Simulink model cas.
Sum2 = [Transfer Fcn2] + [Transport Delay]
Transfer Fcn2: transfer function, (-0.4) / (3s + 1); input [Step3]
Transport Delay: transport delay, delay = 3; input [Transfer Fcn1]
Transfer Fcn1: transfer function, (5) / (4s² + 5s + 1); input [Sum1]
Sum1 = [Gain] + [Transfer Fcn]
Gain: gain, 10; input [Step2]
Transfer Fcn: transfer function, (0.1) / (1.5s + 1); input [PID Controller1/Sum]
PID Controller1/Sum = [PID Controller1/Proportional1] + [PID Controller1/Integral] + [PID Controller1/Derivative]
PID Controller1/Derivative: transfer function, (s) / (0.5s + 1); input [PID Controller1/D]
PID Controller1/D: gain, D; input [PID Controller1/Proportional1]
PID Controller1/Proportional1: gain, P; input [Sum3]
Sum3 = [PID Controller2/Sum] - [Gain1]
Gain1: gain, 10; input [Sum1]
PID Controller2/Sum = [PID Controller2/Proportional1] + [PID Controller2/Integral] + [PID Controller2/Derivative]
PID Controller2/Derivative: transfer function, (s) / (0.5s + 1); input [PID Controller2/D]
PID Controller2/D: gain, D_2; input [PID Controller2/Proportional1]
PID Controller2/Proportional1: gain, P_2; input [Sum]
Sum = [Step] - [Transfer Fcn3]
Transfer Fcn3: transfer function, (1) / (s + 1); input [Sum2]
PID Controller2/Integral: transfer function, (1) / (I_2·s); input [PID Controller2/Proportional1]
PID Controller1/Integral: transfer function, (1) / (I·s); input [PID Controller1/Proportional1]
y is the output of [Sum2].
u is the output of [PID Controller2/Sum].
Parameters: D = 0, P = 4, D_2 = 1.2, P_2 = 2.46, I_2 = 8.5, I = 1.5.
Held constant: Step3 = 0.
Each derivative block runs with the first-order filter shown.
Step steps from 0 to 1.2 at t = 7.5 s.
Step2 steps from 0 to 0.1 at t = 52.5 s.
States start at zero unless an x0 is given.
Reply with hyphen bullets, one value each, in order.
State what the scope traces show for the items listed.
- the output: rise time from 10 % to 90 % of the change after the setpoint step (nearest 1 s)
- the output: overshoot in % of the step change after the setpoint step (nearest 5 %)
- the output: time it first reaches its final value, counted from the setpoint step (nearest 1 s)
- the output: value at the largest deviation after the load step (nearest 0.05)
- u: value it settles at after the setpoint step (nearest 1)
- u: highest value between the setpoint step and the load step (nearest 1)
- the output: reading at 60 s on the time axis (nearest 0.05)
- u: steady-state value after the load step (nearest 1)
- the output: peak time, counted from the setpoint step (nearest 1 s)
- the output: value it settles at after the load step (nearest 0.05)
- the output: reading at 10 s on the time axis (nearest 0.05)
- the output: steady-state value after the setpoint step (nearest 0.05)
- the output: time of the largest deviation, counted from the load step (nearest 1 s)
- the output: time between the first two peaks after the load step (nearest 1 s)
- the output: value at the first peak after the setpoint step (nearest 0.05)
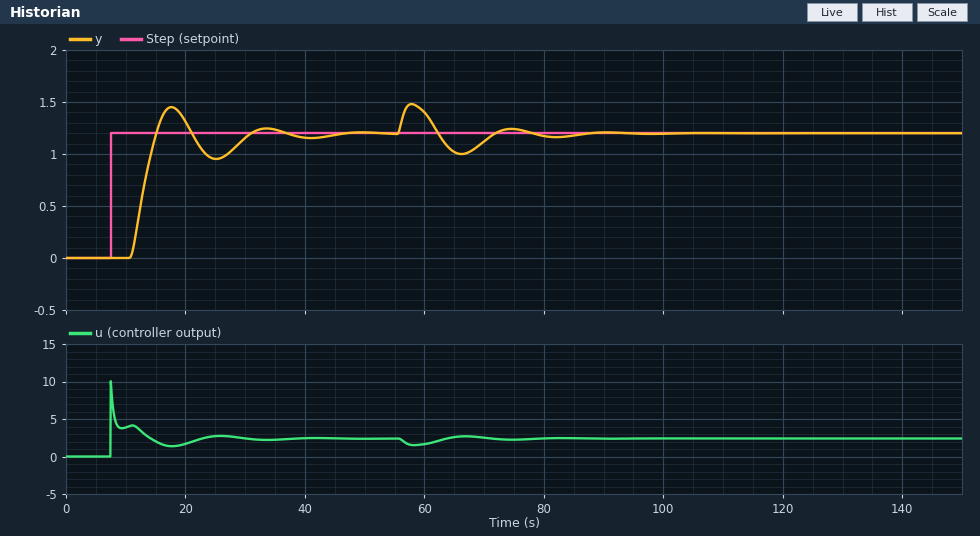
- 3 s
- 20 %
- 8 s
- 1.50
- 2
- 10
- 1.40
- 2
- 10 s
- 1.20
- 0.00
- 1.20
- 5 s
- 17 s
- 1.45
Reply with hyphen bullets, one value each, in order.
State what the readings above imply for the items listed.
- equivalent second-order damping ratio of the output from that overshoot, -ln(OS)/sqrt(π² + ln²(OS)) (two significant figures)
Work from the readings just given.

- 0.46
